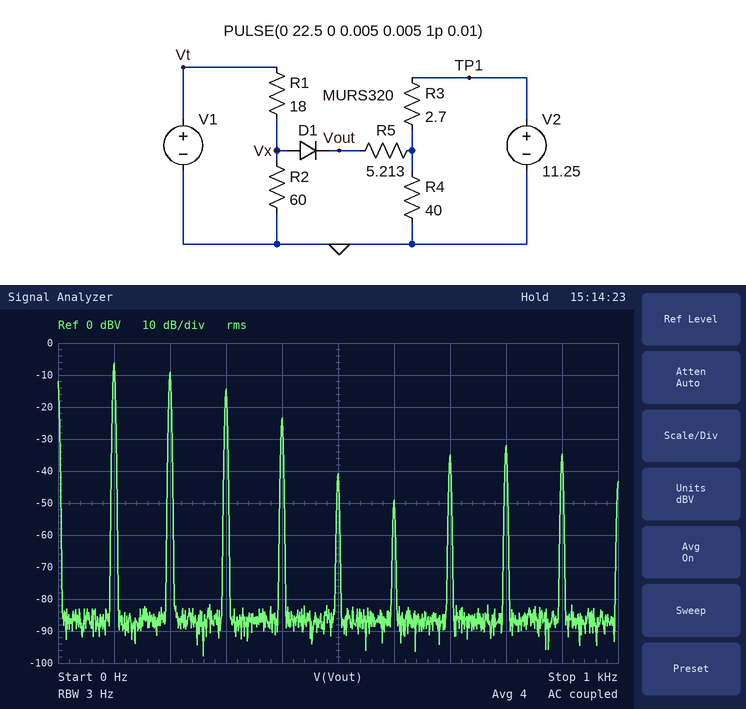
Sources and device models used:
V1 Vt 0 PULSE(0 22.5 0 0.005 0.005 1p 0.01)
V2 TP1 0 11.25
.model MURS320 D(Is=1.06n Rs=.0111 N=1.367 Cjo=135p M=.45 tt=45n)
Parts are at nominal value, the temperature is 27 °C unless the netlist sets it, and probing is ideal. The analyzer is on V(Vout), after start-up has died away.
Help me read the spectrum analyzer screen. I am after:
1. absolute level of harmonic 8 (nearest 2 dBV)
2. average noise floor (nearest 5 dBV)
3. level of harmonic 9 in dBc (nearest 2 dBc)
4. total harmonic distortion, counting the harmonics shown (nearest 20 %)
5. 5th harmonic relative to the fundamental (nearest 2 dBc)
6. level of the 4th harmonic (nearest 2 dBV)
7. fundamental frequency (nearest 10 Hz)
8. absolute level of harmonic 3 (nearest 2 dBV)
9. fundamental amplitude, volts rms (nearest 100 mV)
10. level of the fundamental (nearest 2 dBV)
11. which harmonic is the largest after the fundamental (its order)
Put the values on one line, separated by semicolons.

-32 dBV; -85 dBV; -28 dBc; 80 %; -34 dBc; -24 dBV; 100 Hz; -14 dBV; 500 mV; -6 dBV; 2
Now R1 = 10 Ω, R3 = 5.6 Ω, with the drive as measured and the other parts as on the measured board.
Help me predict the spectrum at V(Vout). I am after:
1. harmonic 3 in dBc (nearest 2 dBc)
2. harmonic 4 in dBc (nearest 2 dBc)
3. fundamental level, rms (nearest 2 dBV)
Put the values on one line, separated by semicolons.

-14 dBc; -38 dBc; 2 dBV
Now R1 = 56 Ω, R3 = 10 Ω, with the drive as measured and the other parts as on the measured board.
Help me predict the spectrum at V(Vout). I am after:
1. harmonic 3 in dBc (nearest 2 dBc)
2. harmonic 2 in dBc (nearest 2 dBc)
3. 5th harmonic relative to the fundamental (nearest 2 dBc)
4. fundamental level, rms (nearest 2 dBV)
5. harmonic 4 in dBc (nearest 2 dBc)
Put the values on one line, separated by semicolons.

-2 dBc; 0 dBc; -6 dBc; -22 dBV; -4 dBc
